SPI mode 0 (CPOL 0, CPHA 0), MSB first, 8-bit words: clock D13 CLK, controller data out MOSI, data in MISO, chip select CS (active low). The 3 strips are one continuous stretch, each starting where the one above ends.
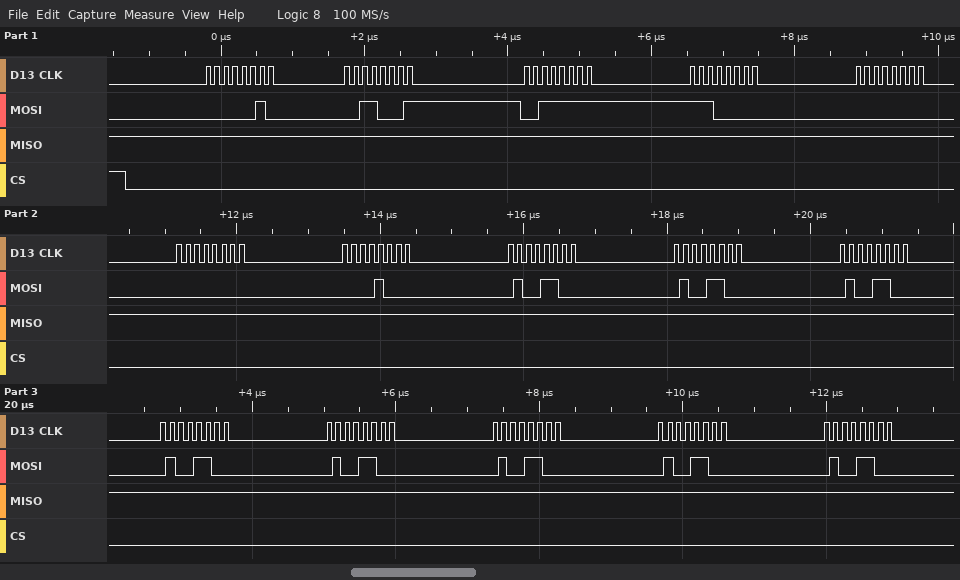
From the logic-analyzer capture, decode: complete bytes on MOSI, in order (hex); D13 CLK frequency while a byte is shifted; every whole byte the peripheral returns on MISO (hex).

02 31 3F E0 00 00 08 4C 4C 4C 4C 4C 4C 4C 4C
8 MHz
FF FF FF FF FF FF FF FF FF FF FF FF FF FF FF
